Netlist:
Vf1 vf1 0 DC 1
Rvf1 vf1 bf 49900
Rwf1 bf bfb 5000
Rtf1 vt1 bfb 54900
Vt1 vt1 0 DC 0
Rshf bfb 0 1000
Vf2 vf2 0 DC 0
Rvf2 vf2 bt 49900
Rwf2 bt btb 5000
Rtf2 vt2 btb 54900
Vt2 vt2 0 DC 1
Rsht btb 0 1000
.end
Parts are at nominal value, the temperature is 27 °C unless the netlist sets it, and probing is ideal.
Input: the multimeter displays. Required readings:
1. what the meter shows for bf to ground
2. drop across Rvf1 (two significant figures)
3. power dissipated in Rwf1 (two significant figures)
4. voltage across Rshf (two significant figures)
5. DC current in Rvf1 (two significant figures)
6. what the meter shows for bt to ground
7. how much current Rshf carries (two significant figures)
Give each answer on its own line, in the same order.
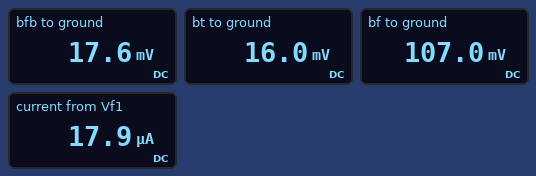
107.0 mV
890 mV
1.6 µW
18 mV
18 µA
16.0 mV
18 µA
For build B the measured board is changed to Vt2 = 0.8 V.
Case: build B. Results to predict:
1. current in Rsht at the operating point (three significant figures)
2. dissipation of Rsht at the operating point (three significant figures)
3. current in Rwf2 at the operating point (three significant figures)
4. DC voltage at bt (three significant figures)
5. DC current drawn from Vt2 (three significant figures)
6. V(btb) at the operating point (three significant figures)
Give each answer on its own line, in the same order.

14.1 µA
198 nW
256 nA
12.8 mV
14.3 µA
14.1 mV
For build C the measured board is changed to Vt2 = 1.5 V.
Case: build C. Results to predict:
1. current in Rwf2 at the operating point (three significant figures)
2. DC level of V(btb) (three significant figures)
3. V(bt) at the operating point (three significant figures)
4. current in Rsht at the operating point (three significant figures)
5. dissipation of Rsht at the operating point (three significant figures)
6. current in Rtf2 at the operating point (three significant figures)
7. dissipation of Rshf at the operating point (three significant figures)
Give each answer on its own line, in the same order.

480 nA
26.4 mV
24.0 mV
26.4 µA
695 nW
26.8 µA
309 nW
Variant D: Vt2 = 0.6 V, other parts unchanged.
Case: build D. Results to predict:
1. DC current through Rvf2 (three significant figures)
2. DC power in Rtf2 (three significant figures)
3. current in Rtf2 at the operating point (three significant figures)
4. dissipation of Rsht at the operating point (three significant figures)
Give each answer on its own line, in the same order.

192 nA
6.33 µW
10.7 µA
111 nW
